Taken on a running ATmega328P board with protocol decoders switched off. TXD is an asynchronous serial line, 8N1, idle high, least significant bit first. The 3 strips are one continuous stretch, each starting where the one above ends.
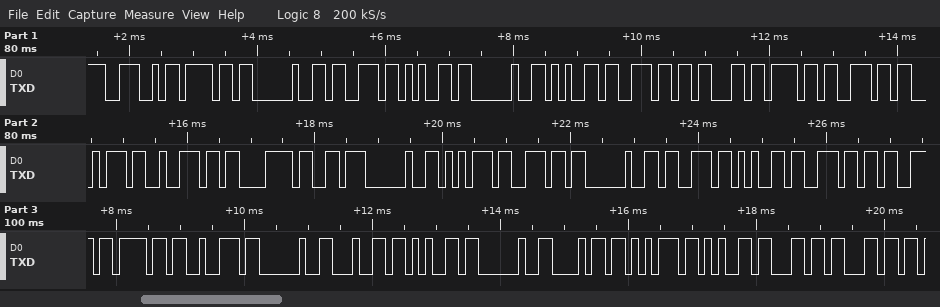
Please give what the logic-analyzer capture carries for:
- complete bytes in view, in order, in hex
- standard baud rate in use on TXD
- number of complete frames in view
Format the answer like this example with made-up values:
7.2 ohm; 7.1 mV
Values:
4E 6F 20 73 65 20 65 6E 63 6F 6E 74 72 C3 B3 20 75 6E 20 73 65 6E 73 6F 72 20 64 65 20 68 75 65 6C 6C; 9600 baud; 34
